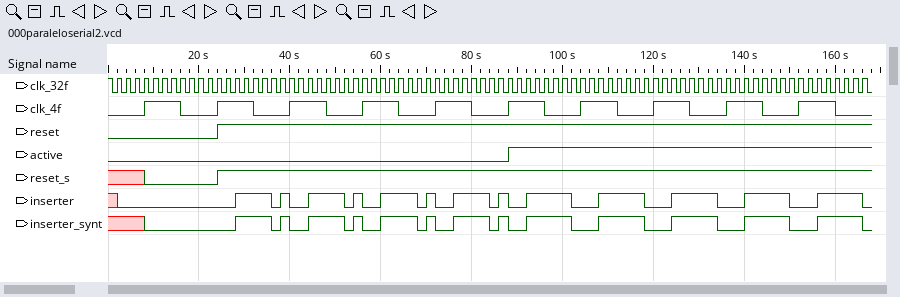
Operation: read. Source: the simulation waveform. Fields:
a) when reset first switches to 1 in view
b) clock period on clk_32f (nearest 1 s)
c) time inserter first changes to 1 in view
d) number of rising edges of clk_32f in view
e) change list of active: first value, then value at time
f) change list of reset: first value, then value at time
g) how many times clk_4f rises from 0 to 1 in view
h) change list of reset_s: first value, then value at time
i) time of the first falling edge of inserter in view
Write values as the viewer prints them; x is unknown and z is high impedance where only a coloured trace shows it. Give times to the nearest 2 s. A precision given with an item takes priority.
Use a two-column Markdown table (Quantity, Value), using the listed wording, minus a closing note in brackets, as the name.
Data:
| Quantity | Value |
|---|---|
| when reset first switches to 1 in view | 24 s |
| clock period on clk_32f | 2 s |
| time inserter first changes to 1 in view | 28 s |
| number of rising edges of clk_32f in view | 83 |
| change list of active: first value, then value at time | 0, 1 at 88 s |
| change list of reset: first value, then value at time | 0, 1 at 24 s |
| how many times clk_4f rises from 0 to 1 in view | 10 |
| change list of reset_s: first value, then value at time | x, 0 at 8 s, 1 at 24 s |
| time of the first falling edge of inserter in view | 36 s |
